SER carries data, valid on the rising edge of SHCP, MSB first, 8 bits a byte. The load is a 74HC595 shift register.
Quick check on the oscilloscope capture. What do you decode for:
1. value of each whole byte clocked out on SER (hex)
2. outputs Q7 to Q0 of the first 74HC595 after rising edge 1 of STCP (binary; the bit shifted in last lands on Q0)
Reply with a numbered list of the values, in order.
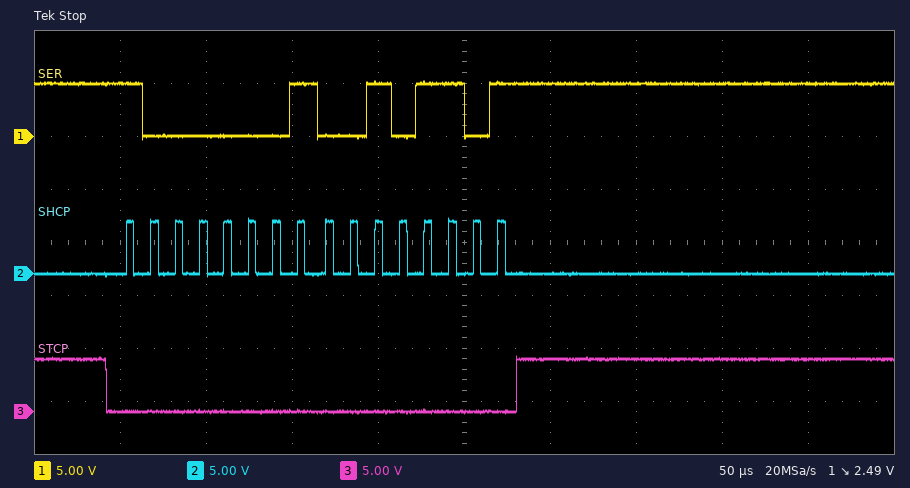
1. 81 2D
2. 00101101
